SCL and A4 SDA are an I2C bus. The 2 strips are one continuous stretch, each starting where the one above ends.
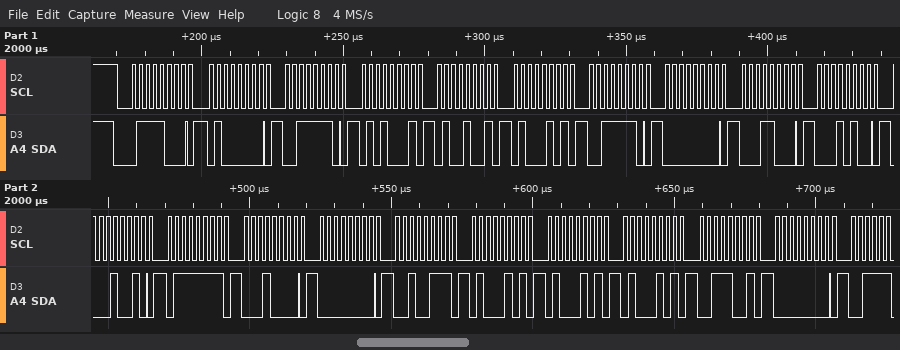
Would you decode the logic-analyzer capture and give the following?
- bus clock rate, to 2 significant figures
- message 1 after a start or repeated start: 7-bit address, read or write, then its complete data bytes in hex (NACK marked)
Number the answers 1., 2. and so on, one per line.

1. 400 kHz
2. 0x3C write: 40 3E 51 49 45 3E 00 18 14 12 7F 10 00 27 45 45 45 39 00
